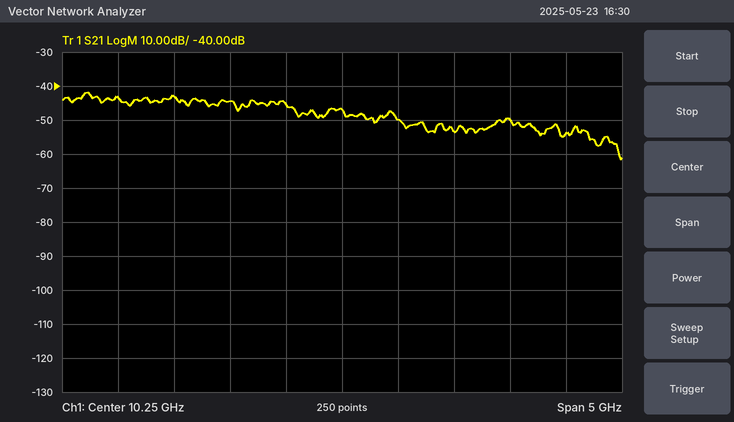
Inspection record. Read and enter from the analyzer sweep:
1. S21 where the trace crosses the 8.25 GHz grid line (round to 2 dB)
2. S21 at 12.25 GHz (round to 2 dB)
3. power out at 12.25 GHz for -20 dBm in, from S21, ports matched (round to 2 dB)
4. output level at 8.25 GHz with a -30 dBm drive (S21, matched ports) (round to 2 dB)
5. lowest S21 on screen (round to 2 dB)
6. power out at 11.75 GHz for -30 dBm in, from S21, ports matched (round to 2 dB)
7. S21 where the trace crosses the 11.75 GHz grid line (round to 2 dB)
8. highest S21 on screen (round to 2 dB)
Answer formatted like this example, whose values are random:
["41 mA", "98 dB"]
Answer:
["-44 dB", "-54 dB", "-74 dBm", "-74 dBm", "-62 dB", "-80 dBm", "-50 dB", "-42 dB"]
